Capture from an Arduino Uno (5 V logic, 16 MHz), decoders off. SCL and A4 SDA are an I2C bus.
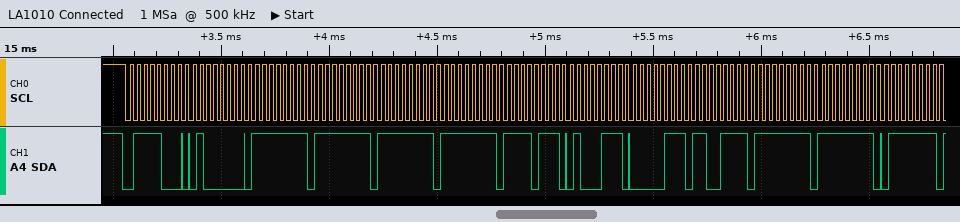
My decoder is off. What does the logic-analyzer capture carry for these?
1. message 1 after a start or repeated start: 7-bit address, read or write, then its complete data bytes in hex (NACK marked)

0x3C write: 40 FF FF FF FF F7 47 07 CF FF FF 7F
